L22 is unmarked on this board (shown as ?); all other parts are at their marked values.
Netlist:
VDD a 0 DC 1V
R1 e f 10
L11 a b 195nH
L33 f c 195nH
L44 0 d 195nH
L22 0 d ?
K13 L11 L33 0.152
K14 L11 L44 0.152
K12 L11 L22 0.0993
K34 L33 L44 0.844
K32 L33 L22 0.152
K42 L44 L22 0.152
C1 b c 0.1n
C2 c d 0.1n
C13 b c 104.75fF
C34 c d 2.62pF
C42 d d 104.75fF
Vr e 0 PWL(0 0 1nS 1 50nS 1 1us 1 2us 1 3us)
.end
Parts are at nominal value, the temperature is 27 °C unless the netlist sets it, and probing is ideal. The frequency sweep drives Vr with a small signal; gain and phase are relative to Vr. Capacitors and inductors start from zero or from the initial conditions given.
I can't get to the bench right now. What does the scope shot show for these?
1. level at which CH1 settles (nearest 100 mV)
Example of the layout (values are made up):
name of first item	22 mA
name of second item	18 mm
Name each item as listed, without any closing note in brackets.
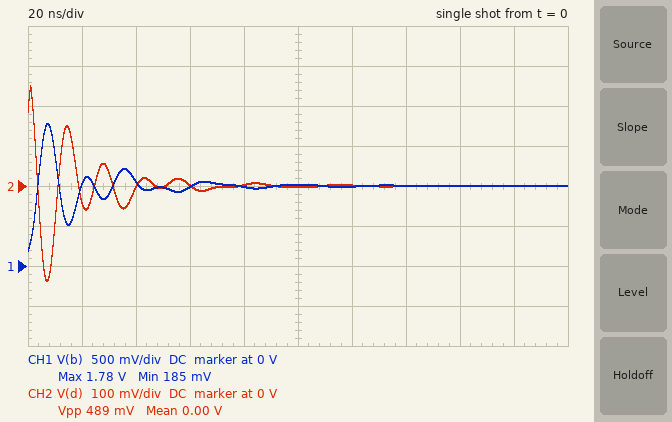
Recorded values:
level at which CH1 settles	1.0 V
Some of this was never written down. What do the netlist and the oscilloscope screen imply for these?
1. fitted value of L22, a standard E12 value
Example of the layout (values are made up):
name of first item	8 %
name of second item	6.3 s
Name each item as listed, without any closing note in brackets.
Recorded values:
fitted value of L22, a standard E12 value	68 nH
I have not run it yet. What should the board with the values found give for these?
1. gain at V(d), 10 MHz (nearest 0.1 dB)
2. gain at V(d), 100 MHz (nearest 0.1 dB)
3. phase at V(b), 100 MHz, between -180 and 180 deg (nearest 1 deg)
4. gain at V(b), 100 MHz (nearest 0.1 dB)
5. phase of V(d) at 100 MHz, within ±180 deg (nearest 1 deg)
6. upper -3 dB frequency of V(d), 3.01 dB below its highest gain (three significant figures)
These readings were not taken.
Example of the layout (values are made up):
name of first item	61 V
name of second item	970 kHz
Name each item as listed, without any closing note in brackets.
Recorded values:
gain at V(d), 10 MHz	-38.0 dB
gain at V(d), 100 MHz	-10.3 dB
phase at V(b), 100 MHz, between -180 and 180 deg	-153 deg
gain at V(b), 100 MHz	-5.3 dB
phase of V(d) at 100 MHz, within ±180 deg	27 deg
upper -3 dB frequency of V(d), 3.01 dB below its highest gain	81.0 MHz
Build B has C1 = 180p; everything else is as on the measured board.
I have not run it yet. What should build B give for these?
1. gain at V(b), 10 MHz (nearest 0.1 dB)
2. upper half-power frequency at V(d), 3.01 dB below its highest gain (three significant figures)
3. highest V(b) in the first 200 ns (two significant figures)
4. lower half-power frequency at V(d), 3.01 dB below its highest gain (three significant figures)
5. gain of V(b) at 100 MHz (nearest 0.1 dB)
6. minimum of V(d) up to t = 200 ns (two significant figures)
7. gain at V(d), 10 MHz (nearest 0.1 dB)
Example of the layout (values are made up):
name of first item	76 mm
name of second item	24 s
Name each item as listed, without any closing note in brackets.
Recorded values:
gain at V(b), 10 MHz	-16.4 dB
upper half-power frequency at V(d), 3.01 dB below its highest gain	81.4 MHz
highest V(b) in the first 200 ns	1.7 V
lower half-power frequency at V(d), 3.01 dB below its highest gain	60.2 MHz
gain of V(b) at 100 MHz	-5.8 dB
minimum of V(d) up to t = 200 ns	-220 mV
gain at V(d), 10 MHz	-31.3 dB
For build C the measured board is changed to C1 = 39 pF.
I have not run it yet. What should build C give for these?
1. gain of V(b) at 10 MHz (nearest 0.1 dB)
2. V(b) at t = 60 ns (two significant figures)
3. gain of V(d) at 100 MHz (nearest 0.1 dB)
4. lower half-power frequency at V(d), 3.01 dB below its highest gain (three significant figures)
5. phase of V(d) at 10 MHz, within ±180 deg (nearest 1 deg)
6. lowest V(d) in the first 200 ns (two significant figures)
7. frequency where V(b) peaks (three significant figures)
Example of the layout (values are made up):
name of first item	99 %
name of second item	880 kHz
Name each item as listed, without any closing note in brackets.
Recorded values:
gain of V(b) at 10 MHz	-31.2 dB
V(b) at t = 60 ns	1.1 V
gain of V(d) at 100 MHz	-9.3 dB
lower half-power frequency at V(d), 3.01 dB below its highest gain	67.2 MHz
phase of V(d) at 10 MHz, within ±180 deg	-5 deg
lowest V(d) in the first 200 ns	-270 mV
frequency where V(b) peaks	73.4 MHz
